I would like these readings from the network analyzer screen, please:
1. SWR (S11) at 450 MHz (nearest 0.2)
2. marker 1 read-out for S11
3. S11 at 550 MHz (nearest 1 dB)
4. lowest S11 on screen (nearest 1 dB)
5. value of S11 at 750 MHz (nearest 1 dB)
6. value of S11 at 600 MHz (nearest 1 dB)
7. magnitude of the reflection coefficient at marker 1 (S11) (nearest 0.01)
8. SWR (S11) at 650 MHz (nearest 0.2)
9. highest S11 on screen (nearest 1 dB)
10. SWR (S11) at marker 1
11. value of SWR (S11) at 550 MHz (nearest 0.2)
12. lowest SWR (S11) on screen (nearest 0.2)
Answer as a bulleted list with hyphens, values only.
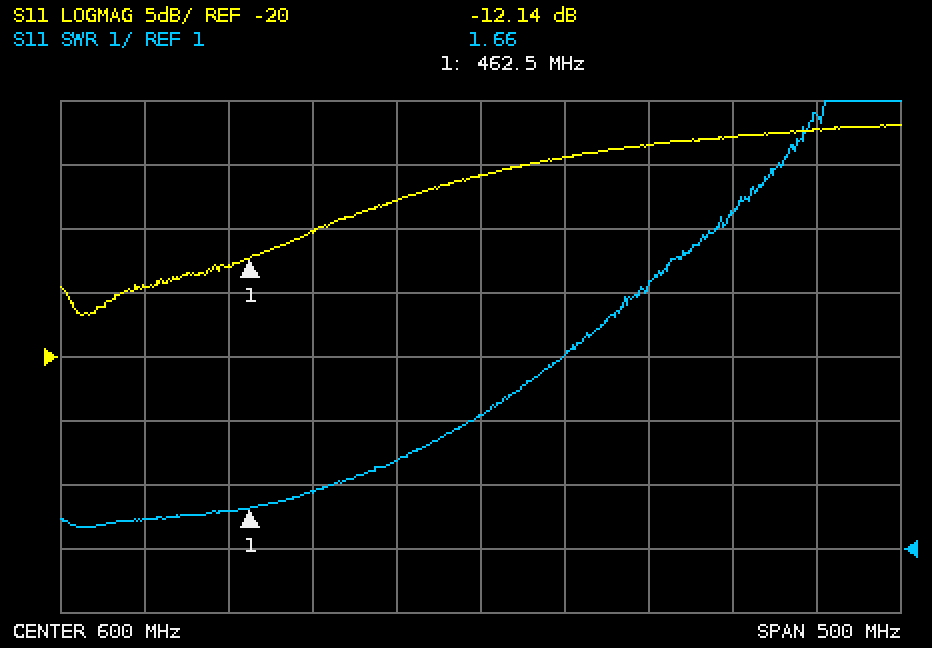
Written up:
- 1.6
- -12.14 dB
- -8 dB
- -17 dB
- -3 dB
- -6 dB
- 0.25
- 4.0
- -2 dB
- 1.66
- 2.4
- 1.4
